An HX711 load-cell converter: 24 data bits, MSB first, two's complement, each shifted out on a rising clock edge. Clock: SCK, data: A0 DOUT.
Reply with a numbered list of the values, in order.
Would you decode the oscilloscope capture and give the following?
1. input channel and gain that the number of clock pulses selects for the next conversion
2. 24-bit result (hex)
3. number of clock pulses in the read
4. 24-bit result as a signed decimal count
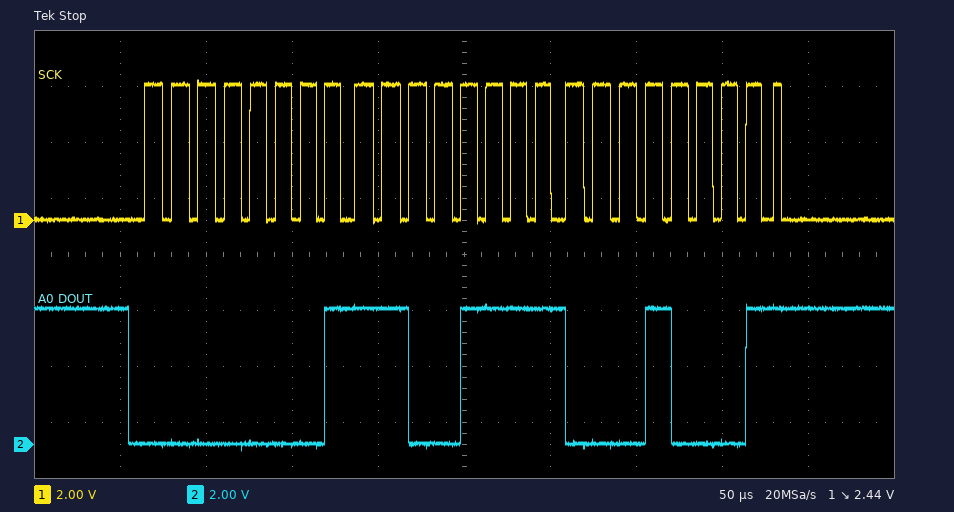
1. channel A, gain 128
2. 0x01CF11
3. 25
4. 118545
